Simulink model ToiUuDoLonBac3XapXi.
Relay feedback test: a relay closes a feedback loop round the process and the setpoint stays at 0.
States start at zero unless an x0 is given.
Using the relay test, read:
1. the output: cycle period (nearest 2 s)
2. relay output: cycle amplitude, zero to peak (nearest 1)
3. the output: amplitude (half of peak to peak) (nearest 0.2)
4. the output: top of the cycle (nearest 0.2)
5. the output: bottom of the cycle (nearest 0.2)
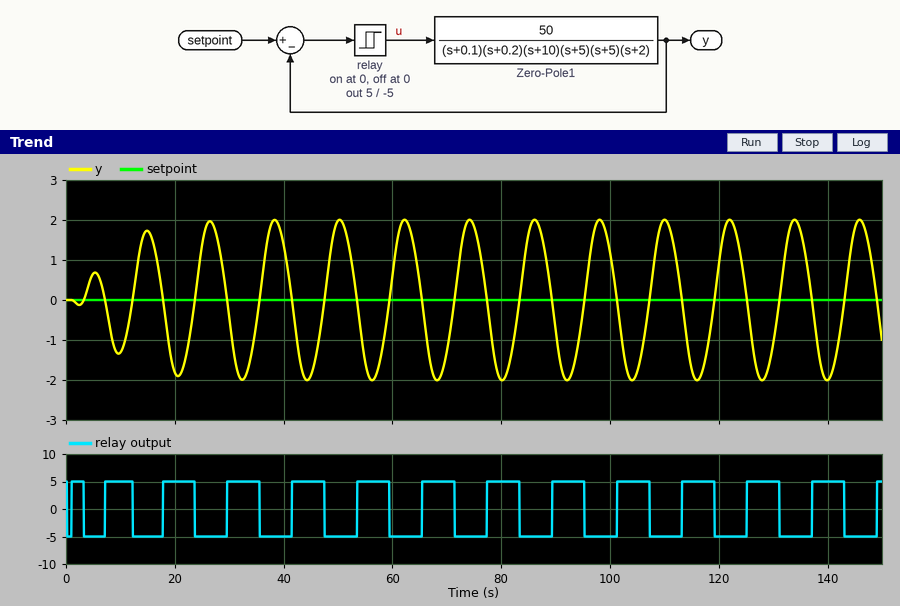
12 s
5
2.0
2.0
-2.0
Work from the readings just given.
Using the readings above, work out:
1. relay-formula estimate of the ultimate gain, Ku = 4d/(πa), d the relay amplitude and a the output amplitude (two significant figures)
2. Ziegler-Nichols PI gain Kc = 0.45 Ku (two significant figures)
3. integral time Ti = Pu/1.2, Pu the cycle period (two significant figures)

3.2
1.4
10 s
